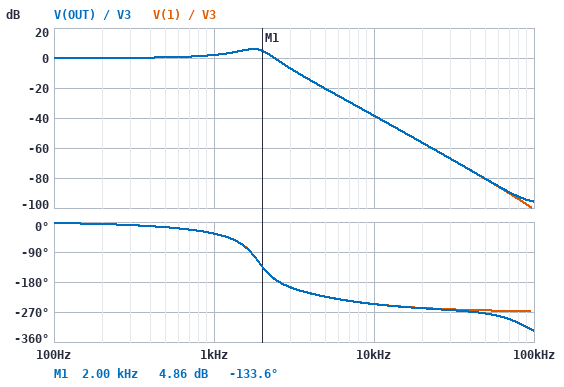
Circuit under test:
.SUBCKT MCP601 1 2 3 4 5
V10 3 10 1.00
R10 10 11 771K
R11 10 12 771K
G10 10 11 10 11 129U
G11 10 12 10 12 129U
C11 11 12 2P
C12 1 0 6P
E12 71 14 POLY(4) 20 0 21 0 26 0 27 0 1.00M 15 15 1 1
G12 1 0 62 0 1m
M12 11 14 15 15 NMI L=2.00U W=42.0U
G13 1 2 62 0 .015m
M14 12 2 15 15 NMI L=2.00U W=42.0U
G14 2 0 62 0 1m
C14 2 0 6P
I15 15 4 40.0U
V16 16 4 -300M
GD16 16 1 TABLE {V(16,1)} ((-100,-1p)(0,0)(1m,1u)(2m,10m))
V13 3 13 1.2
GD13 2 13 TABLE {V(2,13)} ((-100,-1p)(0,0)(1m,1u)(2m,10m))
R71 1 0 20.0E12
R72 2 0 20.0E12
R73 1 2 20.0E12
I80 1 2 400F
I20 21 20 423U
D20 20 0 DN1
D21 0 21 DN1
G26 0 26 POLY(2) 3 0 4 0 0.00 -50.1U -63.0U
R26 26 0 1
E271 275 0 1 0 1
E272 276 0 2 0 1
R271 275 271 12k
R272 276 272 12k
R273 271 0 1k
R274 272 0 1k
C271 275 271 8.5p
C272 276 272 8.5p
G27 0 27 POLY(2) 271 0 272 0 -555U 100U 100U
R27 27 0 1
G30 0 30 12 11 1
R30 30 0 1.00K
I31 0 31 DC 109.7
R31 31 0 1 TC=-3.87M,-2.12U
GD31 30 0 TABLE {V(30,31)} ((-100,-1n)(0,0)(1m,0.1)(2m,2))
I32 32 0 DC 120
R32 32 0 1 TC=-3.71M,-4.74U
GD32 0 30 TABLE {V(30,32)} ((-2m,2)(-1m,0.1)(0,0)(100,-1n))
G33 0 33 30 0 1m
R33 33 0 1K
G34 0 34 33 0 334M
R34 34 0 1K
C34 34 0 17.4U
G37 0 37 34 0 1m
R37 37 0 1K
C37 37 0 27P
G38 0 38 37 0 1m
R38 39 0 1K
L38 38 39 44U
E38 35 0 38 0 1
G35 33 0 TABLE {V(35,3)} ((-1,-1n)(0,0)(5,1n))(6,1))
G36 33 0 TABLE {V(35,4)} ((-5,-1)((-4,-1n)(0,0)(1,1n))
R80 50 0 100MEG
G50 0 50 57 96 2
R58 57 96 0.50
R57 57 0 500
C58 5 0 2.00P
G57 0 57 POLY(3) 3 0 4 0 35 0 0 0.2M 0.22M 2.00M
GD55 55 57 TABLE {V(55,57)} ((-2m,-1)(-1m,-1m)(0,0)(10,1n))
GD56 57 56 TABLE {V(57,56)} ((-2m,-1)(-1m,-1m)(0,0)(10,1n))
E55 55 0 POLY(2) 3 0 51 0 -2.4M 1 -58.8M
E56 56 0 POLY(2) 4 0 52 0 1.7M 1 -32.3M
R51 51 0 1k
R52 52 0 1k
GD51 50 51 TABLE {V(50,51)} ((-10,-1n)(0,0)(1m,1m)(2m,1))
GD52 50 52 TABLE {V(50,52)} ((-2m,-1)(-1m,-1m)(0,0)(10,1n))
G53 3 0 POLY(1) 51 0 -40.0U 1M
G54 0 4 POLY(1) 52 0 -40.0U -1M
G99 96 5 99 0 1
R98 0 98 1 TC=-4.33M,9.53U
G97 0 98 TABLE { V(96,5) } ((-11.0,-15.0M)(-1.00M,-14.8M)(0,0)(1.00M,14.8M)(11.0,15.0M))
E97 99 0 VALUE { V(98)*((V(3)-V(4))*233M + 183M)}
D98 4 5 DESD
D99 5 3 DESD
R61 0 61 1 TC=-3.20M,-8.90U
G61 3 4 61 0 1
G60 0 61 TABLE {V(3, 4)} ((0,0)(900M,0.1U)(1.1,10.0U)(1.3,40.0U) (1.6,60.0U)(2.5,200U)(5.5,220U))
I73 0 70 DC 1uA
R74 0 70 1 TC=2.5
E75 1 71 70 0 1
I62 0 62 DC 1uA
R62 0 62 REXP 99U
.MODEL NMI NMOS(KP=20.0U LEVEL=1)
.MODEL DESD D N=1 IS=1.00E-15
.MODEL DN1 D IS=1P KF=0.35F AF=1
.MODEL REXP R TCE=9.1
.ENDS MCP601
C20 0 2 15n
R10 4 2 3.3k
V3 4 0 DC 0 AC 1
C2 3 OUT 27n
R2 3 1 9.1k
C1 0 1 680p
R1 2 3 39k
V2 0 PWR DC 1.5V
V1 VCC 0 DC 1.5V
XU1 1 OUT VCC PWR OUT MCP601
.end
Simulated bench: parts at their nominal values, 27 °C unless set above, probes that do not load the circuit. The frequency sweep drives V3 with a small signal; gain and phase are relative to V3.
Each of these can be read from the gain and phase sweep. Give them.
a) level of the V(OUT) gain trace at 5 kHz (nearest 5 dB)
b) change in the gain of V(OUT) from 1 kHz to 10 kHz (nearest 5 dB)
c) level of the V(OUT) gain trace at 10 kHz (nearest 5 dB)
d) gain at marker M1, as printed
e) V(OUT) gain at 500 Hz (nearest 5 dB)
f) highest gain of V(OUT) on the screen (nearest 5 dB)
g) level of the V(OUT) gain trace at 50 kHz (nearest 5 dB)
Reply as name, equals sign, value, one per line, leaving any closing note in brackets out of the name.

level of the V(OUT) gain trace at 5 kHz = -20 dB
change in the gain of V(OUT) from 1 kHz to 10 kHz = -40 dB
level of the V(OUT) gain trace at 10 kHz = -40 dB
gain at marker M1, as printed = 4.86 dB
V(OUT) gain at 500 Hz = 0 dB
highest gain of V(OUT) on the screen = 5 dB
level of the V(OUT) gain trace at 50 kHz = -80 dB
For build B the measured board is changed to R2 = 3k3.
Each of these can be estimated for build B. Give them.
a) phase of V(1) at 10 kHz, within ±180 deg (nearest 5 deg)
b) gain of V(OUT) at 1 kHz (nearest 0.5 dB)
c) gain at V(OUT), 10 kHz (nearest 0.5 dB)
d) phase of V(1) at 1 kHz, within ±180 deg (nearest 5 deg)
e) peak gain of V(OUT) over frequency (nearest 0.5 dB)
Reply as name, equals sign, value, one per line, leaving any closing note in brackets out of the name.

phase of V(1) at 10 kHz, within ±180 deg = 120 deg
gain of V(OUT) at 1 kHz = 0.5 dB
gain at V(OUT), 10 kHz = -29.5 dB
phase of V(1) at 1 kHz, within ±180 deg = -30 deg
peak gain of V(OUT) over frequency = 2.0 dB
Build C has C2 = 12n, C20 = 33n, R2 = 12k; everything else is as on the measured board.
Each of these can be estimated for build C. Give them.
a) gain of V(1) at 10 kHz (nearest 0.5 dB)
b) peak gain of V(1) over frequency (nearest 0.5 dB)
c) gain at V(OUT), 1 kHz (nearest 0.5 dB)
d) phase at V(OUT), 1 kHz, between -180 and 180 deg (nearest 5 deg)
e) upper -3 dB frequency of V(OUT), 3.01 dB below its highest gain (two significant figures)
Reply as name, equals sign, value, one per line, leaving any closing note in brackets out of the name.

gain of V(1) at 10 kHz = -40.0 dB
peak gain of V(1) over frequency = 0 dB
gain at V(OUT), 1 kHz = -0.5 dB
phase at V(OUT), 1 kHz, between -180 and 180 deg = -50 deg
upper -3 dB frequency of V(OUT), 3.01 dB below its highest gain = 2.7 kHz
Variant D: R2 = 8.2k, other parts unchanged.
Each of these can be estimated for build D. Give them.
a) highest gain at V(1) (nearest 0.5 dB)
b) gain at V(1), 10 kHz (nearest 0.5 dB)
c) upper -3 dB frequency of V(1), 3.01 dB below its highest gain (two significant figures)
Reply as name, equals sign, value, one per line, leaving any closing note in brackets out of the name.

highest gain at V(1) = 5.5 dB
gain at V(1), 10 kHz = -37.5 dB
upper -3 dB frequency of V(1), 3.01 dB below its highest gain = 2.3 kHz
